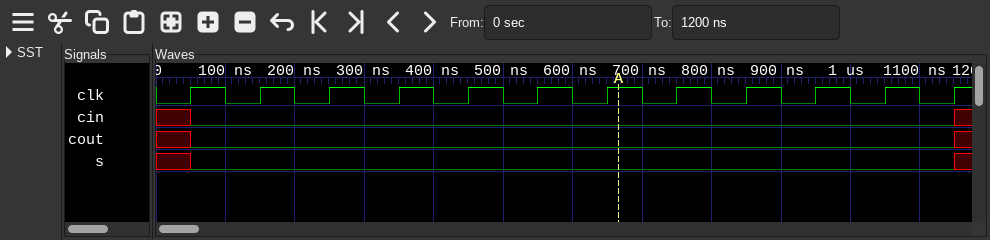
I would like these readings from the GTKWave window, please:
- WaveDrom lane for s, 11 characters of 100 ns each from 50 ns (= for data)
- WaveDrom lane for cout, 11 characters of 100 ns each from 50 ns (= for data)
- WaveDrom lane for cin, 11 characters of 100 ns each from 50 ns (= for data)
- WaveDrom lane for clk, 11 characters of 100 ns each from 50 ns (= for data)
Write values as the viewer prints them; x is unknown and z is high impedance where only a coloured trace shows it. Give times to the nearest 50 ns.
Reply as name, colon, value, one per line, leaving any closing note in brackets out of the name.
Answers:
WaveDrom lane for s, 11 characters of 100 ns each from 50 ns: {name: 's', wave: '0..........'}
WaveDrom lane for cout, 11 characters of 100 ns each from 50 ns: {name: 'cout', wave: '0..........'}
WaveDrom lane for cin, 11 characters of 100 ns each from 50 ns: {name: 'cin', wave: '0..........'}
WaveDrom lane for clk, 11 characters of 100 ns each from 50 ns: {name: 'clk', wave: 'p..........'}
